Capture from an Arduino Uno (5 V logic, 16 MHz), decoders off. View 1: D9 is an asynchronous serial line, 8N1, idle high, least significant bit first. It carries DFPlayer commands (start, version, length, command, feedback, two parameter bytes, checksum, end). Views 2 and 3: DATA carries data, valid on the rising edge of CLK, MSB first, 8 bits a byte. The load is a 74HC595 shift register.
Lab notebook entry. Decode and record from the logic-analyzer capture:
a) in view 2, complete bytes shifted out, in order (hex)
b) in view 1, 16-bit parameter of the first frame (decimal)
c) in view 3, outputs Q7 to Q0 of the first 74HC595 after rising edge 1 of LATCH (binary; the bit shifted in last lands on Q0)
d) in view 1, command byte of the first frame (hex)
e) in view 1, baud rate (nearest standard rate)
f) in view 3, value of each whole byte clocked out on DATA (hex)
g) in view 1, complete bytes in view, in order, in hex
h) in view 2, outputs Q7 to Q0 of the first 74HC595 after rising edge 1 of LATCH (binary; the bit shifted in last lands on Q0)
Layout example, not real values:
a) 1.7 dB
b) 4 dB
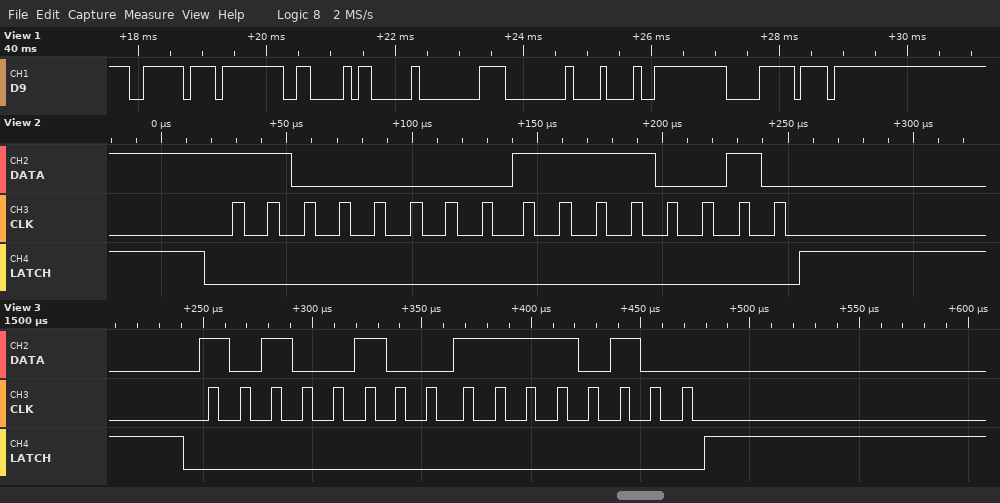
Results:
a) C0 F2
b) 8
c) 11110100
d) 0x03
e) 9600 baud
f) A4 F4
g) 7E FF 06 03 00 00 08 FE F0 EF
h) 11110010
